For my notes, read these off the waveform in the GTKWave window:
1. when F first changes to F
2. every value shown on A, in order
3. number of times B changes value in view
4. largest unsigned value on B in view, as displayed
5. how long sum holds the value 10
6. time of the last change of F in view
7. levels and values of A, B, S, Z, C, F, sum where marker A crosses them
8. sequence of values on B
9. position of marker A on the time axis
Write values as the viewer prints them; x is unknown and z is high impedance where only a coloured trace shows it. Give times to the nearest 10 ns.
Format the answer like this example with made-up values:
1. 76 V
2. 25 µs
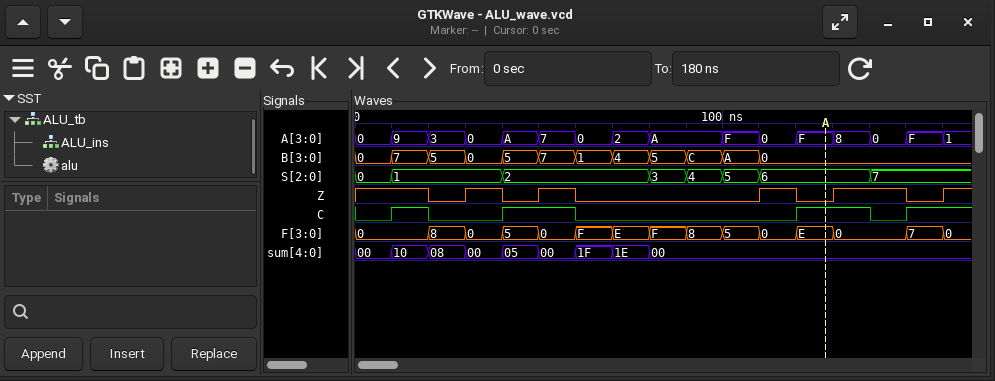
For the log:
1. 60 ns
2. 0, 9, 3, 0, A, 7, 0, 2, A, F, 0, F, 8, 0, F, 1
3. 11
4. C
5. 10 ns
6. 160 ns
7. A=F, B=0, S=6, Z=0, C=1, F=E, sum=00
8. 0, 7, 5, 0, 5, 7, 1, 4, 5, C, A, 0
9. 130 ns
